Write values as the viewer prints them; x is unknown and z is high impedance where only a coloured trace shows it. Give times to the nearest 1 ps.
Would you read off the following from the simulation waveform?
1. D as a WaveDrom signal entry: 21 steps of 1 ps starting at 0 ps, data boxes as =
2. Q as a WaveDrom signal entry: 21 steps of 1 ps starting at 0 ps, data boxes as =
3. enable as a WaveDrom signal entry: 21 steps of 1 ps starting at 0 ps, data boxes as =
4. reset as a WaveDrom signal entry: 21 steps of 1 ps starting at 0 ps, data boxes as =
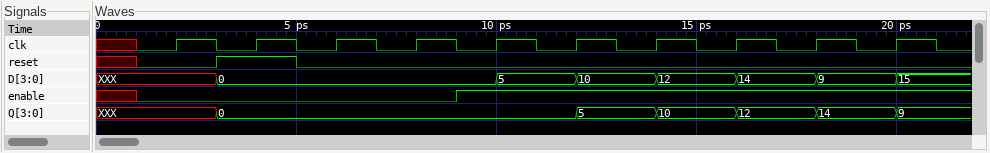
{name: 'D', wave: 'x..=......=.=.=.=.=.=', data: '0 5 10 12 14 9 15'}
{name: 'Q', wave: 'x..=........=.=.=.=.=', data: '0 5 10 12 14 9'}
{name: 'enable', wave: 'x0.......1...........'}
{name: 'reset', wave: 'x0.1.0...............'}
